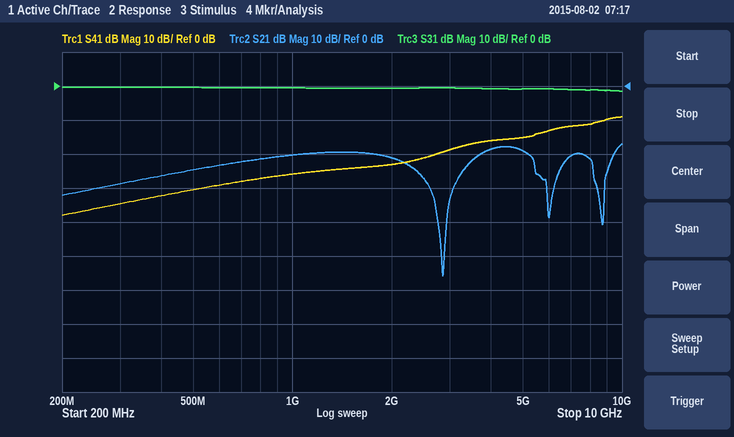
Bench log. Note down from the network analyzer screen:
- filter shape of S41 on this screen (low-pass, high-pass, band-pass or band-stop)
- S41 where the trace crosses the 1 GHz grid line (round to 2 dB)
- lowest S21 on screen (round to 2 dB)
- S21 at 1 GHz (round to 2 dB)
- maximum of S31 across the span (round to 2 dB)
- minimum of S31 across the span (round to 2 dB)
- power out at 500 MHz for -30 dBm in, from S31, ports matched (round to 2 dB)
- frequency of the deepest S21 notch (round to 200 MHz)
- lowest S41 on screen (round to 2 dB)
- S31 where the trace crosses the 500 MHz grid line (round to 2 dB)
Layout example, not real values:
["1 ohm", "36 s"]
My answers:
["high-pass", "-26 dB", "-56 dB", "-20 dB", "0 dB", "-2 dB", "-30 dBm", "2.8 GHz", "-38 dB", "0 dB"]
